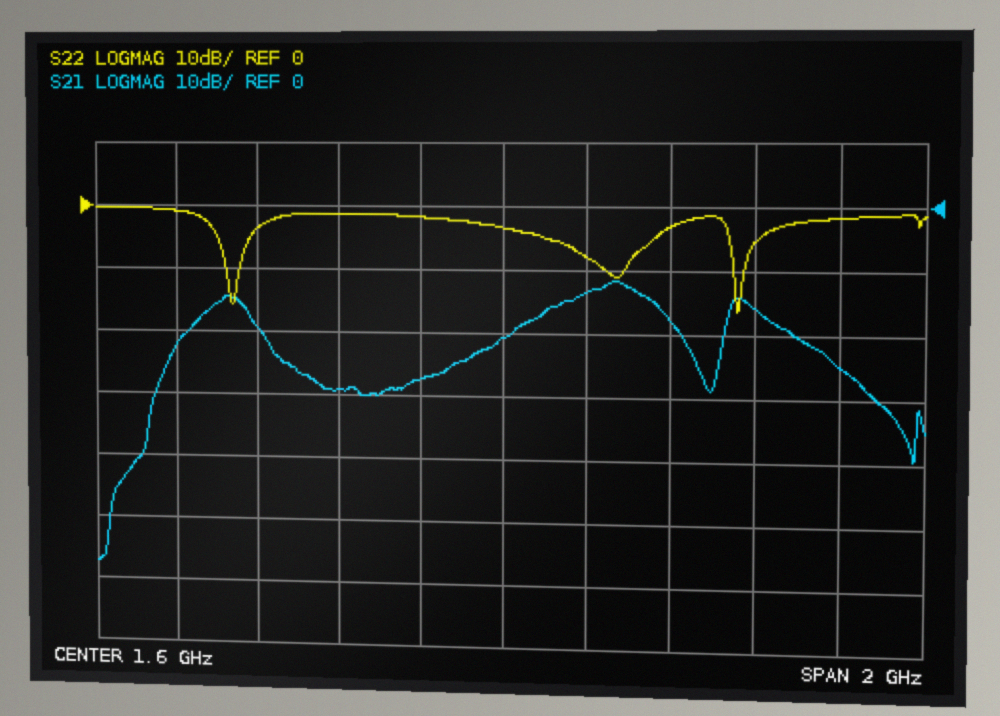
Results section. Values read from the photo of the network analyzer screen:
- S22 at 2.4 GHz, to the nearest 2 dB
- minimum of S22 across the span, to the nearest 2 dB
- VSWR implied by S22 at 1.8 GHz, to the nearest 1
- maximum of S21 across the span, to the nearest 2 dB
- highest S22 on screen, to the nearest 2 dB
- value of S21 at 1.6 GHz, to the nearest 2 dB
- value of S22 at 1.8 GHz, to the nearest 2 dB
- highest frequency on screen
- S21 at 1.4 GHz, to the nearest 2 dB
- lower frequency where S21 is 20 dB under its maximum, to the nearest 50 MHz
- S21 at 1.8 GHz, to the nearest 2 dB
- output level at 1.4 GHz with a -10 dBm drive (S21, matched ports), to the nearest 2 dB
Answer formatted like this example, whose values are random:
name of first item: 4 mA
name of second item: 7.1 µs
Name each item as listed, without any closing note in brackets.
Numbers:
S22 at 2.4 GHz, to the nearest 2 dB: -2 dB
minimum of S22 across the span, to the nearest 2 dB: -16 dB
VSWR implied by S22 at 1.8 GHz, to the nearest 1: 2
maximum of S21 across the span, to the nearest 2 dB: -12 dB
highest S22 on screen, to the nearest 2 dB: 0 dB
value of S21 at 1.6 GHz, to the nearest 2 dB: -20 dB
value of S22 at 1.8 GHz, to the nearest 2 dB: -8 dB
highest frequency on screen: 2.6 GHz
S21 at 1.4 GHz, to the nearest 2 dB: -28 dB
lower frequency where S21 is 20 dB under its maximum, to the nearest 50 MHz: 750 MHz
S21 at 1.8 GHz, to the nearest 2 dB: -14 dB
output level at 1.4 GHz with a -10 dBm drive (S21, matched ports), to the nearest 2 dB: -38 dBm
